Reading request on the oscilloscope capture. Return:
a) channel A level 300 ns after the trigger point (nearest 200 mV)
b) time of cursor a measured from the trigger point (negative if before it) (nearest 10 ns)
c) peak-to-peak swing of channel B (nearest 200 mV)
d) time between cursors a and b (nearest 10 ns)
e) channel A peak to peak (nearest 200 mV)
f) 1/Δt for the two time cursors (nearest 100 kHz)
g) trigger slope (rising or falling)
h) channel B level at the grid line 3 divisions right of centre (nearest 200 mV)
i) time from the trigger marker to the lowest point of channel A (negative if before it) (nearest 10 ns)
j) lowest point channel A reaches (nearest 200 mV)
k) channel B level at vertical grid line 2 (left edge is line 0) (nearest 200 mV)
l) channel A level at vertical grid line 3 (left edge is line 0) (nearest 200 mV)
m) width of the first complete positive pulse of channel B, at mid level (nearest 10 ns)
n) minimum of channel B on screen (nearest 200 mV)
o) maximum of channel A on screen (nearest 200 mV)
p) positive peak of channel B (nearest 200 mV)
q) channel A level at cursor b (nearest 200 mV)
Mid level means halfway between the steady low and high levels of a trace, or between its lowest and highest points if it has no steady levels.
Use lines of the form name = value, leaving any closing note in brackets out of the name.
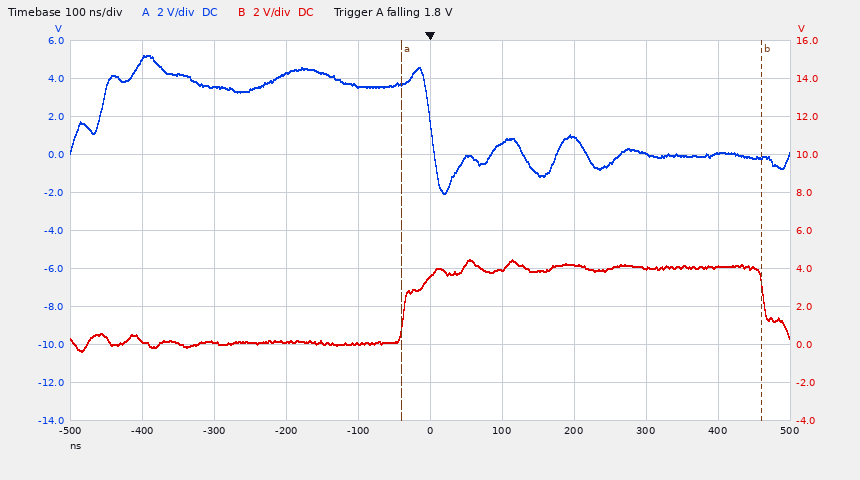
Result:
channel A level 300 ns after the trigger point = 0.0 V
time of cursor a measured from the trigger point (negative if before it) = -40 ns
peak-to-peak swing of channel B = 4.8 V
time between cursors a and b = 500 ns
channel A peak to peak = 7.2 V
1/Δt for the two time cursors = 2.0 MHz
trigger slope = falling
channel B level at the grid line 3 divisions right of centre = 4.0 V
time from the trigger marker to the lowest point of channel A (negative if before it) = +20 ns
lowest point channel A reaches = -2.0 V
channel B level at vertical grid line 2 (left edge is line 0) = 200 mV
channel A level at vertical grid line 3 (left edge is line 0) = 4.2 V
width of the first complete positive pulse of channel B, at mid level = 500 ns
minimum of channel B on screen = -400 mV
maximum of channel A on screen = 5.2 V
positive peak of channel B = 4.4 V
channel A level at cursor b = -200 mV
